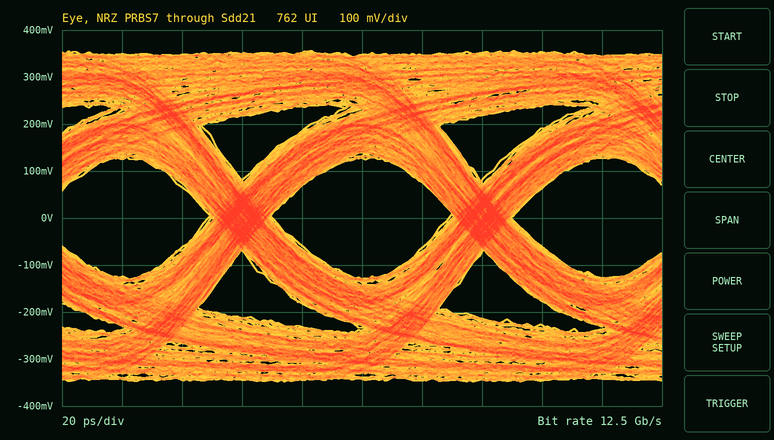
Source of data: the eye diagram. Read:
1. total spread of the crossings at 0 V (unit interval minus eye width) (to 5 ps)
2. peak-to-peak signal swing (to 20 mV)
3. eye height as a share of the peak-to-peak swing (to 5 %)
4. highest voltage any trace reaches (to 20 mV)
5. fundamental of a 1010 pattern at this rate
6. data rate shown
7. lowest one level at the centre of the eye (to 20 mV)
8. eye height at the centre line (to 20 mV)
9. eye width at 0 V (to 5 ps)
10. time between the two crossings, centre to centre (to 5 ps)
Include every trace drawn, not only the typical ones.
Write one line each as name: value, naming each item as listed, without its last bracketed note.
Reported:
total spread of the crossings at 0 V (unit interval minus eye width): 20 ps
peak-to-peak signal swing: 700 mV
eye height as a share of the peak-to-peak swing: 35 %
highest voltage any trace reaches: 360 mV
fundamental of a 1010 pattern at this rate: 6.25 GHz
data rate shown: 12.5 Gb/s
lowest one level at the centre of the eye: 120 mV
eye height at the centre line: 260 mV
eye width at 0 V: 60 ps
time between the two crossings, centre to centre: 80 ps
